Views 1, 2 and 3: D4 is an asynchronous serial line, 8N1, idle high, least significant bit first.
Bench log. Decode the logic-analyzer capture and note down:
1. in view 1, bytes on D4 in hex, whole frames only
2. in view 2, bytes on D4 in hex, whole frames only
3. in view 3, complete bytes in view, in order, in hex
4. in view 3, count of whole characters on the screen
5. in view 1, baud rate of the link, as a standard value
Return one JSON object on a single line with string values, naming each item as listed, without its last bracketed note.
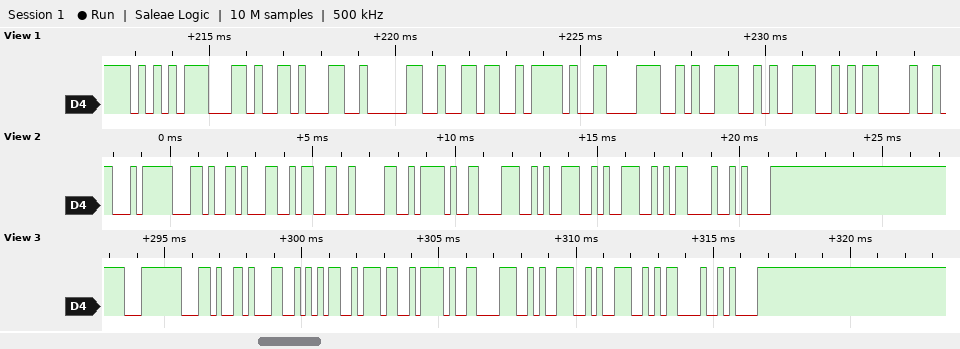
{"in view 1, bytes on D4 in hex, whole frames only": "D5 2C 31 30 36 2F 38 39 39 0D", "in view 2, bytes on D4 in hex, whole frames only": "F4 2C 31 33 30 2F 38 39 39 0D 0A", "in view 3, complete bytes in view, in order, in hex": "FC 2C 31 35 37 2F 38 39 39 0D 0A", "in view 3, count of whole characters on the screen": "11", "in view 1, baud rate of the link, as a standard value": "4800 baud"}
